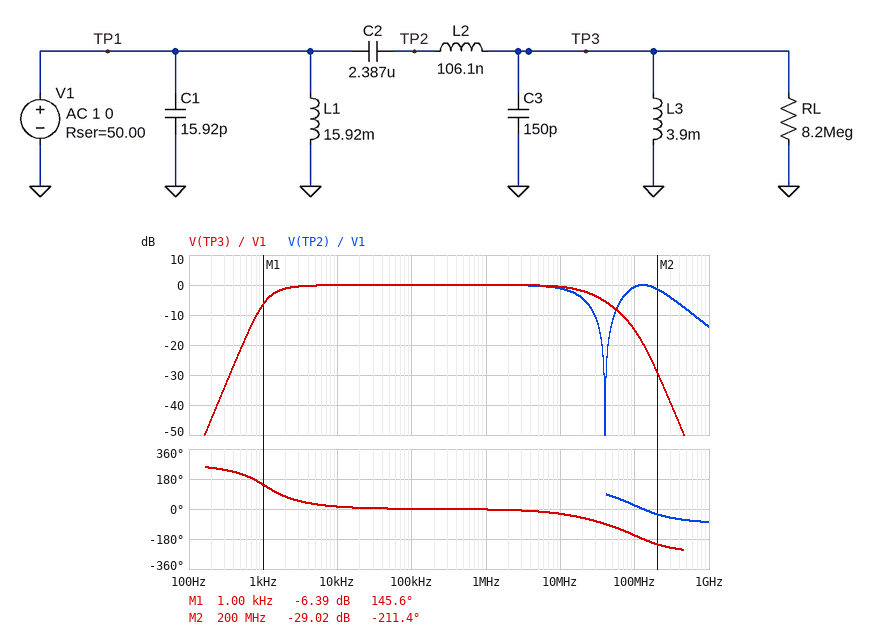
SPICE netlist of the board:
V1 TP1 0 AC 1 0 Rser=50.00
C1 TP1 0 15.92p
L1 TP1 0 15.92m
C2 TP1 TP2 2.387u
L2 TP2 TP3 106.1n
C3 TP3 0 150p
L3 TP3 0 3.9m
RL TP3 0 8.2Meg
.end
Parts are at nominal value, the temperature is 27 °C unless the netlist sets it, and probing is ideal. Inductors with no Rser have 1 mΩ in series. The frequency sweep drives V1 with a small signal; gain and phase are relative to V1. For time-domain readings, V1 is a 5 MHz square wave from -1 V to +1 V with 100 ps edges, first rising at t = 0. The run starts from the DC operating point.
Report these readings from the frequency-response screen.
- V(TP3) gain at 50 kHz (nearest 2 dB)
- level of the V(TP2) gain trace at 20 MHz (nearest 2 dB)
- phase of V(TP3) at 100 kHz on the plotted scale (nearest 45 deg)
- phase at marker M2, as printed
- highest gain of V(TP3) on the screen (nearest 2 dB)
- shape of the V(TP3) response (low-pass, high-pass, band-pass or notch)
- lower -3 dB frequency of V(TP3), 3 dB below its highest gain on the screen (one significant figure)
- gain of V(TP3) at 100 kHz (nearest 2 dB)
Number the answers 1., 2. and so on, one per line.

1. 0 dB
2. -4 dB
3. 0 deg
4. -211.4 deg
5. 0 dB
6. band-pass
7. 1 kHz
8. 0 dB
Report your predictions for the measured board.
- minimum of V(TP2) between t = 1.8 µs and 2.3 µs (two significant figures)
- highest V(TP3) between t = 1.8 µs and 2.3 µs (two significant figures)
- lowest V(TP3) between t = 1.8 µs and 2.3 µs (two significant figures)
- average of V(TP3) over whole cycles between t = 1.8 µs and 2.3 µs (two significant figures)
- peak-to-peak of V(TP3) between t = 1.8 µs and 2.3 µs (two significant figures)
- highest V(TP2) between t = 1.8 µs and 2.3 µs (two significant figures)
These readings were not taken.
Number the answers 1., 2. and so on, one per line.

1. -35 mV
2. 2.0 V
3. -35 mV
4. 970 mV
5. 2.0 V
6. 2.0 V
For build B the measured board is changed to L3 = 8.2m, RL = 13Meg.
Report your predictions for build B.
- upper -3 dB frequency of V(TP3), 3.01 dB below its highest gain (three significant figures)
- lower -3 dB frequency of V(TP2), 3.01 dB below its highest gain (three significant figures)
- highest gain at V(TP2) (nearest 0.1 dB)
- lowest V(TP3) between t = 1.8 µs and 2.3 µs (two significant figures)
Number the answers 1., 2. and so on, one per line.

1. 17.5 MHz
2. 790 Hz
3. 1.4 dB
4. -20 mV
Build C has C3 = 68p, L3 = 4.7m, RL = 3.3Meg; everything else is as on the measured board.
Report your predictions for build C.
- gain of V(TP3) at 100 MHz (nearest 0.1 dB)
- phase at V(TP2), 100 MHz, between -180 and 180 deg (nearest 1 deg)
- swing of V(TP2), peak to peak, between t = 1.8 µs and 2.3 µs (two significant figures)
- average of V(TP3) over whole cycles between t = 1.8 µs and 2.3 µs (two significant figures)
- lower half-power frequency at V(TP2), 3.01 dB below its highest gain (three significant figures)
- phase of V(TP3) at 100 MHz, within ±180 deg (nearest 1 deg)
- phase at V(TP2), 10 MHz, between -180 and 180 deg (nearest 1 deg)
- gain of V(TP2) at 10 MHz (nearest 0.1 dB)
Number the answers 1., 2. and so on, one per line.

1. -6.9 dB
2. 33 deg
3. 2.1 V
4. 970 mV
5. 1.11 kHz
6. -147 deg
7. -15 deg
8. -0.3 dB
